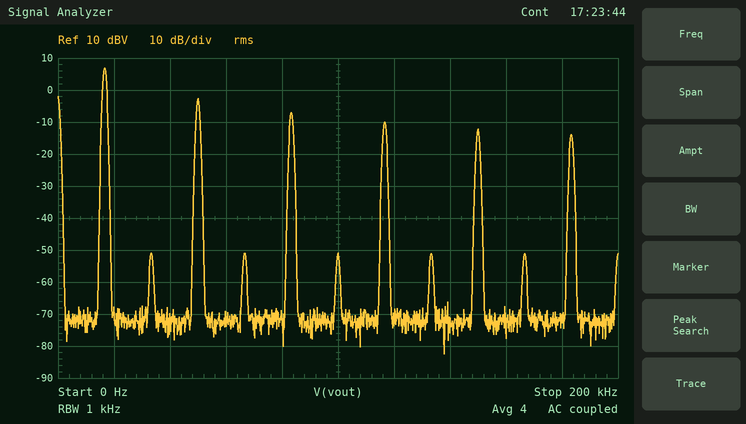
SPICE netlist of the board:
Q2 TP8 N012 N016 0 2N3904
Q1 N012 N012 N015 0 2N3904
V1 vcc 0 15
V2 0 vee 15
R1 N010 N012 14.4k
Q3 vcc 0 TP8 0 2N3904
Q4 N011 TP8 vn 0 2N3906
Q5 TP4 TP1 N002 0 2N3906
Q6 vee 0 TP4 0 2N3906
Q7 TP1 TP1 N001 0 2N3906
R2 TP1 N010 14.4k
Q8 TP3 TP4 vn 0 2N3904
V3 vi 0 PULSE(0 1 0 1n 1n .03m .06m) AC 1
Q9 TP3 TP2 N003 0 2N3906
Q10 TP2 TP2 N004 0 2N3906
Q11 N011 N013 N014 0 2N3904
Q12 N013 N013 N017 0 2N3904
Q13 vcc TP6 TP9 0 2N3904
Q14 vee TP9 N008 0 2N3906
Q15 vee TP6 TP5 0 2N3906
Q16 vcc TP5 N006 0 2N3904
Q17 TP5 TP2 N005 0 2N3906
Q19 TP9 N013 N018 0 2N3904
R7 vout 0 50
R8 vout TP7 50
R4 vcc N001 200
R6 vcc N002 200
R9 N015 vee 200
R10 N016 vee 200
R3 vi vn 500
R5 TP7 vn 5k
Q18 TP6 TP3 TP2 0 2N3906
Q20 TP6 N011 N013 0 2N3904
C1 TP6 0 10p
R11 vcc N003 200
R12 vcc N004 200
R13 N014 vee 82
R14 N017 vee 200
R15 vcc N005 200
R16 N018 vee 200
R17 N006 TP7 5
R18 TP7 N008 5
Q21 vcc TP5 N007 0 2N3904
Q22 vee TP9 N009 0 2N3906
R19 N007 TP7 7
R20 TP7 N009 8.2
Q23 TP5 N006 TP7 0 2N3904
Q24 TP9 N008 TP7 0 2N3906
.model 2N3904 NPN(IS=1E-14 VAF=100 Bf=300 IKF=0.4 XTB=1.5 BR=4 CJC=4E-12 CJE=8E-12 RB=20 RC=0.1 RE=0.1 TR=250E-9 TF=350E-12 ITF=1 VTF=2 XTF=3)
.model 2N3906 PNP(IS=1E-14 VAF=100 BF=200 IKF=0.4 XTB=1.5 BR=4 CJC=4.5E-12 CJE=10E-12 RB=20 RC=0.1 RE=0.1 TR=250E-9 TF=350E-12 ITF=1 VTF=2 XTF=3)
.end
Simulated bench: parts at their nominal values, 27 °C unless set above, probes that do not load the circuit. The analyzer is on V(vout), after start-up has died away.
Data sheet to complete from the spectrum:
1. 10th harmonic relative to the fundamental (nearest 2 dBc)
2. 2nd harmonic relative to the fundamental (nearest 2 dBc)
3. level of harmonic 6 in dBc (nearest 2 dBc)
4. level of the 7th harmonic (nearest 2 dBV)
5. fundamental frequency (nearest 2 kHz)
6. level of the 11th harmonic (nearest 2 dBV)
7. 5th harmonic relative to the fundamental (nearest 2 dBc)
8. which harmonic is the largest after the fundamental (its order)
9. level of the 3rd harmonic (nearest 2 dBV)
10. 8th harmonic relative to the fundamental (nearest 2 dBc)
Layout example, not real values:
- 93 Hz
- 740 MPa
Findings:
- -58 dBc
- -58 dBc
- -58 dBc
- -10 dBV
- 16 kHz
- -14 dBV
- -14 dBc
- 3
- -2 dBV
- -58 dBc
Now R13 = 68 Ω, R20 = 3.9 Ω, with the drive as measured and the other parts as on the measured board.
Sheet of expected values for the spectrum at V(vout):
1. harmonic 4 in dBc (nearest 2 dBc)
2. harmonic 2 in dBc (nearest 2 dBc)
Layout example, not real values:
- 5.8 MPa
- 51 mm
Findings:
- -56 dBc
- -56 dBc
